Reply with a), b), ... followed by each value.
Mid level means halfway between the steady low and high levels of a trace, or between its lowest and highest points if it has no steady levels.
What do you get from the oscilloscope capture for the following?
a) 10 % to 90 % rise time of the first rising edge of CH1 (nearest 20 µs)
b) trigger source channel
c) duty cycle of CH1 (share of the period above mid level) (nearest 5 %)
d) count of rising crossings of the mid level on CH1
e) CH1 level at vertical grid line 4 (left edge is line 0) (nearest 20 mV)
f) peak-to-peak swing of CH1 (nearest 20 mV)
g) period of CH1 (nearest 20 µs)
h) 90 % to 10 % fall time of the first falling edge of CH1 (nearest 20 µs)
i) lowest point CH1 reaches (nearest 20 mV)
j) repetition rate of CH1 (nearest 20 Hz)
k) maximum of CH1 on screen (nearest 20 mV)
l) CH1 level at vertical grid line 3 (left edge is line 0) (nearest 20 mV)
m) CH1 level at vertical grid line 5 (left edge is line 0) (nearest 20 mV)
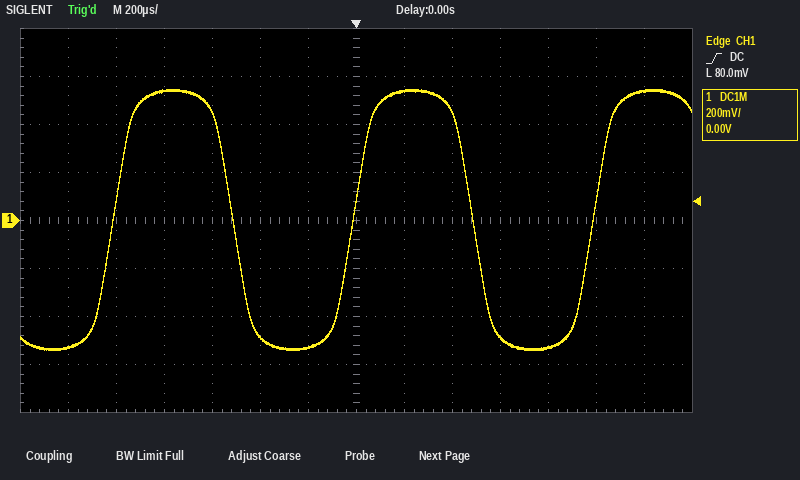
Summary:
a) 160 µs
b) CH1
c) 50 %
d) 3
e) 460 mV
f) 1.08 V
g) 1.00 ms
h) 160 µs
i) -540 mV
j) 1.00 kHz
k) 540 mV
l) 540 mV
m) -480 mV
